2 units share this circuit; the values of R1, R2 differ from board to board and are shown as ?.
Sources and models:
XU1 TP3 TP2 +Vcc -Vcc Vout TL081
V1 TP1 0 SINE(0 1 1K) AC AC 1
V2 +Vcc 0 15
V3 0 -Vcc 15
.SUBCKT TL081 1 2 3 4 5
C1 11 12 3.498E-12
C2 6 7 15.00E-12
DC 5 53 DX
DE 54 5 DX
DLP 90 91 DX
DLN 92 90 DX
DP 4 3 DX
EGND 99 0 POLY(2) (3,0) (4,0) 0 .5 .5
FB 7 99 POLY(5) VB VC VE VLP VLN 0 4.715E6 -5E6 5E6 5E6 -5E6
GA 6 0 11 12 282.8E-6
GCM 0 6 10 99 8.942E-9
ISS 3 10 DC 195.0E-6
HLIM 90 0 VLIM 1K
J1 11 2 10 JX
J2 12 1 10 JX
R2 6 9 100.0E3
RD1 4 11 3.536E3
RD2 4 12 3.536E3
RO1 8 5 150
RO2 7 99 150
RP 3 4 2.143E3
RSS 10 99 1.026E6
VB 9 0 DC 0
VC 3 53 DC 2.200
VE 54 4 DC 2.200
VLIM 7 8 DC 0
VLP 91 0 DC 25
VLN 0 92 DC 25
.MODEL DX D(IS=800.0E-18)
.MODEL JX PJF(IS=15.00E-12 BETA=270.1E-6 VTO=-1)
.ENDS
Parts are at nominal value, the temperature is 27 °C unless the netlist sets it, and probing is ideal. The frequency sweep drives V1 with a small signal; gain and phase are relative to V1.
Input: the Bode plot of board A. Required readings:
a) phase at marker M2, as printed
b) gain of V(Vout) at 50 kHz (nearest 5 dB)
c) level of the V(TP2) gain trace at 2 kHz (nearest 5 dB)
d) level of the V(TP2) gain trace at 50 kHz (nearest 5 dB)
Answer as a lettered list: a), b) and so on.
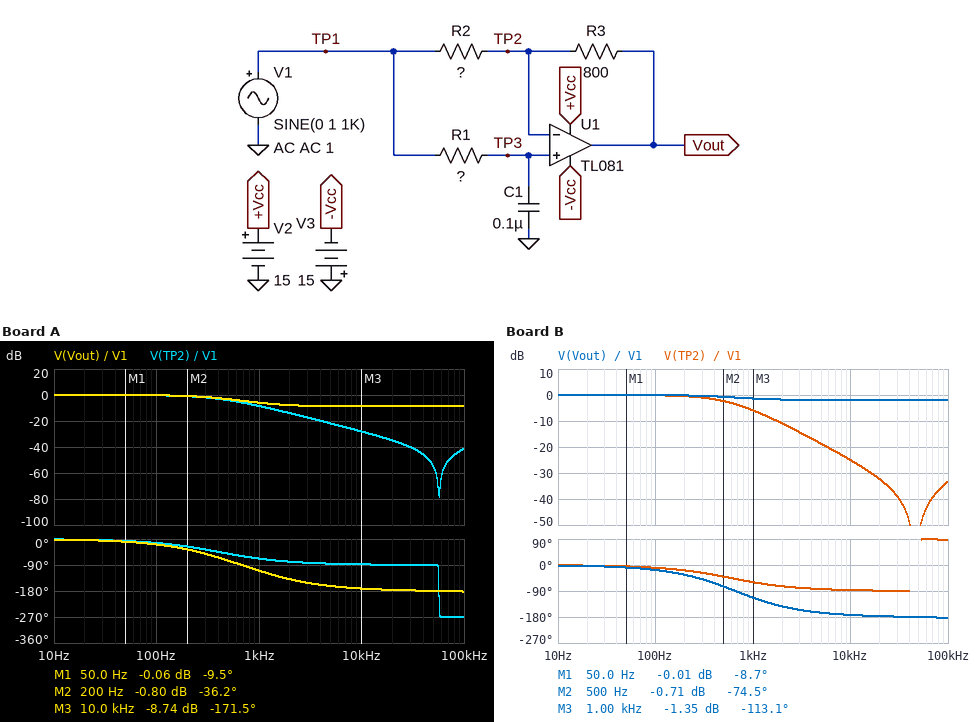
a) -36.2 deg
b) -10 dB
c) -15 dB
d) -55 dB
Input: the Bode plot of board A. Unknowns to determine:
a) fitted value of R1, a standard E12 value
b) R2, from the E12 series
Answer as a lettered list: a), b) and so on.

a) 3.9 kΩ
b) 2.2 kΩ
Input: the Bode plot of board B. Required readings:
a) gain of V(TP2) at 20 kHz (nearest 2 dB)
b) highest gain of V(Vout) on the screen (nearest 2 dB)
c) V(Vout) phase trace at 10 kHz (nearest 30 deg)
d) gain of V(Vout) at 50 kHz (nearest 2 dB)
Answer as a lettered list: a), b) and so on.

a) -32 dB
b) 0 dB
c) -180 deg
d) -2 dB
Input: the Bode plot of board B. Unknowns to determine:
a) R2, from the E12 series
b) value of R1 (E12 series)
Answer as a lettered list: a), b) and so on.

a) 1 kΩ
b) 2.7 kΩ
